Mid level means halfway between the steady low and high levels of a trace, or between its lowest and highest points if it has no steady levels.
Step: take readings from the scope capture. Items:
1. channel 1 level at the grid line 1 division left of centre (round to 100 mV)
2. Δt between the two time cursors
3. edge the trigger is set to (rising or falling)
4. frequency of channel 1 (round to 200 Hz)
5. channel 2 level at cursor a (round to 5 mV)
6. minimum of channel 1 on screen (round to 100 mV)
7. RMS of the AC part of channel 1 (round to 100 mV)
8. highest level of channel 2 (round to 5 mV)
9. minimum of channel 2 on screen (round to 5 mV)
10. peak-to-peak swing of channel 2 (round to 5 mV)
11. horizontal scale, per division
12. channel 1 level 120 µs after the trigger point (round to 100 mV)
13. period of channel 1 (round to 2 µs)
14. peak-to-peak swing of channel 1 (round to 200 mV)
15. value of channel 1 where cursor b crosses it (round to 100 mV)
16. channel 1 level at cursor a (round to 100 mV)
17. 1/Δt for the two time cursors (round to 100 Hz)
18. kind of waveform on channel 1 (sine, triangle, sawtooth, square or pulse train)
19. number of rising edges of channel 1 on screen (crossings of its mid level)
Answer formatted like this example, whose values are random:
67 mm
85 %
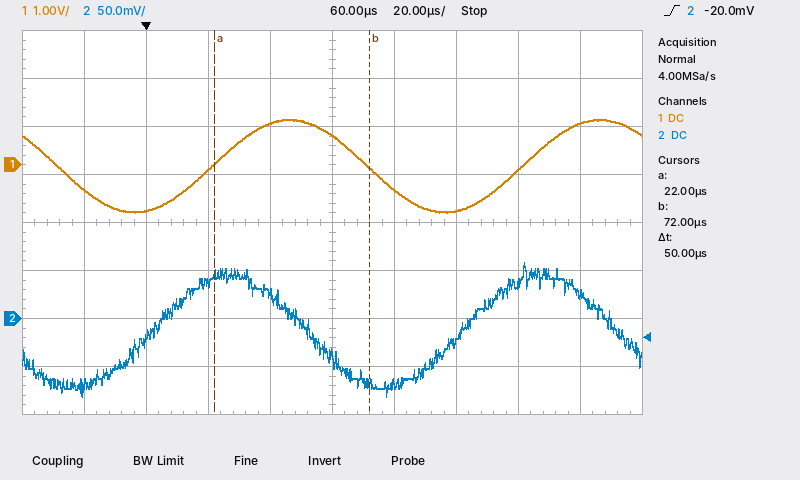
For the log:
900 mV
50 µs
rising
10.0 kHz
45 mV
-1.0 V
700 mV
60 mV
-80 mV
140 mV
20 µs
-100 mV
100 µs
2.0 V
-100 mV
0.0 V
20.0 kHz
sine
2
